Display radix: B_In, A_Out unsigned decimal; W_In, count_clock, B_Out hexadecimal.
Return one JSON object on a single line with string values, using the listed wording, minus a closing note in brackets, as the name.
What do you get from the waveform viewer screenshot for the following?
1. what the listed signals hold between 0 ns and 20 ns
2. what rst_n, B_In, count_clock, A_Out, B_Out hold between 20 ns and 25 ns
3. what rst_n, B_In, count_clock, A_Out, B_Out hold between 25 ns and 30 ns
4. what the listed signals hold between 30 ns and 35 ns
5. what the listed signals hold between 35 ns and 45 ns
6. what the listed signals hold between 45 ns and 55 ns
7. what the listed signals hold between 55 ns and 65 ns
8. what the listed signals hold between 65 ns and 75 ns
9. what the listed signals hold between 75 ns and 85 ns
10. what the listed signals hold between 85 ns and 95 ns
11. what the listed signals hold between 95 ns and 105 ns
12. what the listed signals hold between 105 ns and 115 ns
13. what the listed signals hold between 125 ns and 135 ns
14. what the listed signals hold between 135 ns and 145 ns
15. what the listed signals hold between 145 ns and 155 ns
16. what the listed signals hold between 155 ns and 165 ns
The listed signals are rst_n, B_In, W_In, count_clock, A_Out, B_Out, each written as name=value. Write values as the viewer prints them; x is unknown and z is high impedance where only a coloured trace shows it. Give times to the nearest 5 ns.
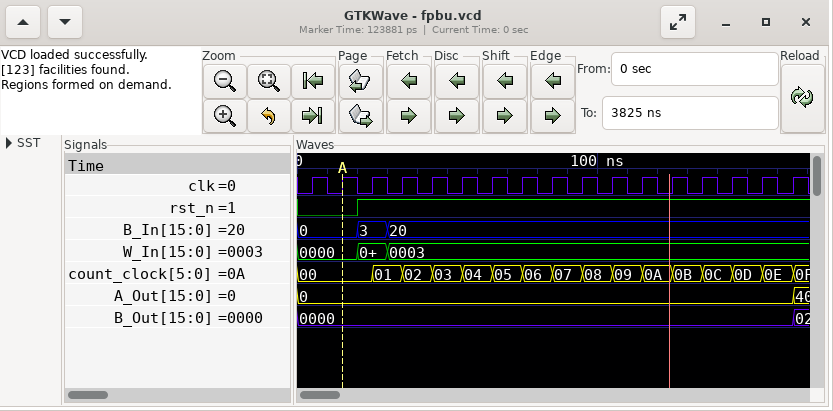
{"what the listed signals hold between 0 ns and 20 ns": "rst_n=0, B_In=0, W_In=0000, count_clock=00, A_Out=0, B_Out=0000", "what rst_n, B_In, count_clock, A_Out, B_Out hold between 20 ns and 25 ns": "rst_n=1, B_In=3, count_clock=00, A_Out=0, B_Out=0000", "what rst_n, B_In, count_clock, A_Out, B_Out hold between 25 ns and 30 ns": "rst_n=1, B_In=3, count_clock=01, A_Out=0, B_Out=0000", "what the listed signals hold between 30 ns and 35 ns": "rst_n=1, B_In=20, W_In=0003, count_clock=01, A_Out=0, B_Out=0000", "what the listed signals hold between 35 ns and 45 ns": "rst_n=1, B_In=20, W_In=0003, count_clock=02, A_Out=0, B_Out=0000", "what the listed signals hold between 45 ns and 55 ns": "rst_n=1, B_In=20, W_In=0003, count_clock=03, A_Out=0, B_Out=0000", "what the listed signals hold between 55 ns and 65 ns": "rst_n=1, B_In=20, W_In=0003, count_clock=04, A_Out=0, B_Out=0000", "what the listed signals hold between 65 ns and 75 ns": "rst_n=1, B_In=20, W_In=0003, count_clock=05, A_Out=0, B_Out=0000", "what the listed signals hold between 75 ns and 85 ns": "rst_n=1, B_In=20, W_In=0003, count_clock=06, A_Out=0, B_Out=0000", "what the listed signals hold between 85 ns and 95 ns": "rst_n=1, B_In=20, W_In=0003, count_clock=07, A_Out=0, B_Out=0000", "what the listed signals hold between 95 ns and 105 ns": "rst_n=1, B_In=20, W_In=0003, count_clock=08, A_Out=0, B_Out=0000", "what the listed signals hold between 105 ns and 115 ns": "rst_n=1, B_In=20, W_In=0003, count_clock=09, A_Out=0, B_Out=0000", "what the listed signals hold between 125 ns and 135 ns": "rst_n=1, B_In=20, W_In=0003, count_clock=0B, A_Out=0, B_Out=0000", "what the listed signals hold between 135 ns and 145 ns": "rst_n=1, B_In=20, W_In=0003, count_clock=0C, A_Out=0, B_Out=0000", "what the listed signals hold between 145 ns and 155 ns": "rst_n=1, B_In=20, W_In=0003, count_clock=0D, A_Out=0, B_Out=0000", "what the listed signals hold between 155 ns and 165 ns": "rst_n=1, B_In=20, W_In=0003, count_clock=0E, A_Out=0, B_Out=0000"}
